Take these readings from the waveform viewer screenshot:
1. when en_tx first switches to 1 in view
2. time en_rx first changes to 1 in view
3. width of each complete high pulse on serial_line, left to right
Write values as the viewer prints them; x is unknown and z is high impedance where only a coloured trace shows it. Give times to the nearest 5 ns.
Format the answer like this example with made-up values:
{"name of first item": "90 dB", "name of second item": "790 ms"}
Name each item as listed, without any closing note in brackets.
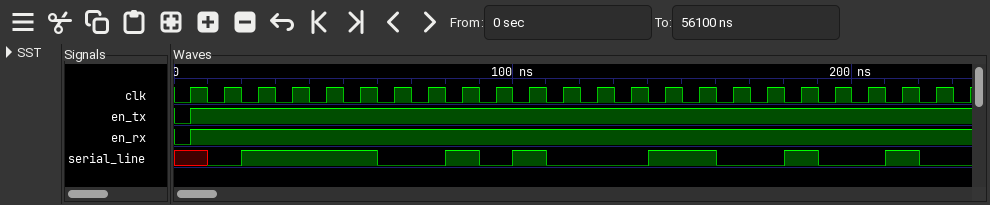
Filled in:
{"when en_tx first switches to 1 in view": "5 ns", "time en_rx first changes to 1 in view": "5 ns", "width of each complete high pulse on serial_line, left to right": "40 ns, 10 ns, 10 ns, 20 ns, 10 ns, 10 ns"}
